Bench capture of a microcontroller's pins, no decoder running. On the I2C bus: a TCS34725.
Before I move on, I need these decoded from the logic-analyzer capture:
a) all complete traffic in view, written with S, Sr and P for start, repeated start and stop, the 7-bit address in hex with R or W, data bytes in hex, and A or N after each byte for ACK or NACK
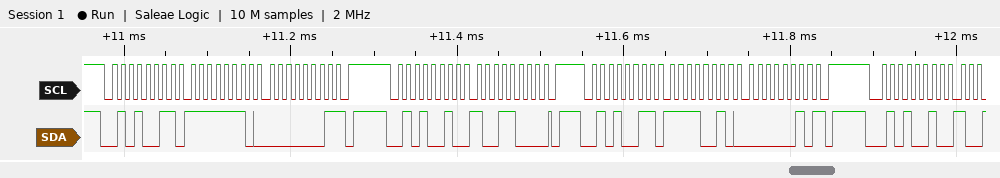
S 29R A FE A 01 N P S 29W A 98 A P S 29R A F2 A 02 N P S 29W A
